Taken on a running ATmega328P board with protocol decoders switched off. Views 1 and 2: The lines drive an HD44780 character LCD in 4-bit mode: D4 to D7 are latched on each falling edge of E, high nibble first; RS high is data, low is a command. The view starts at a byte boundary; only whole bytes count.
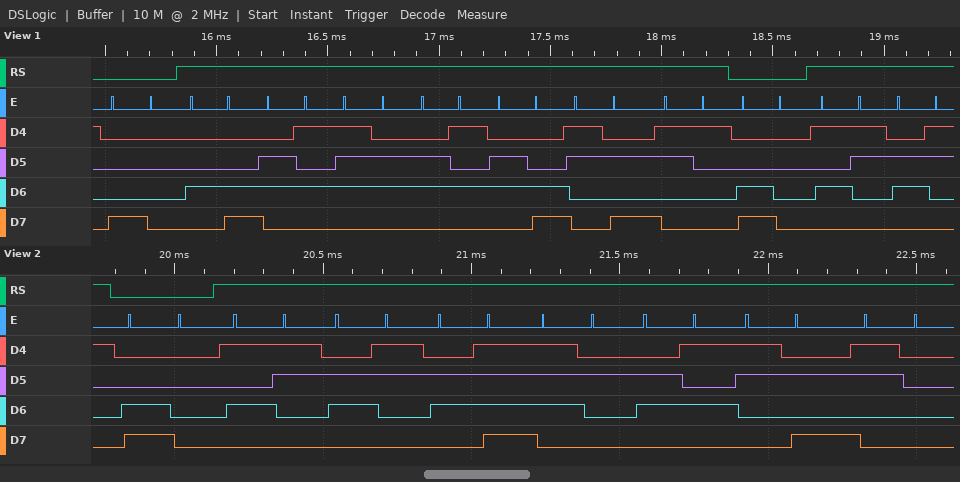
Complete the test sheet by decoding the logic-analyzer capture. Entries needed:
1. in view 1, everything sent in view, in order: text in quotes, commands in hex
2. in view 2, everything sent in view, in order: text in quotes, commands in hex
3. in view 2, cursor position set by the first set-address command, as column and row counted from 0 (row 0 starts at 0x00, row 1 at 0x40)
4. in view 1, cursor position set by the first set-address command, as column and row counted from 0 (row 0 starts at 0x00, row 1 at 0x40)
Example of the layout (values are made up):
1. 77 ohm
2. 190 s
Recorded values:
1. 0x80 "Level:1" 0xC0 "Sc"
2. 0xC0 "Score:0"
3. column 0, row 1
4. column 0, row 0
